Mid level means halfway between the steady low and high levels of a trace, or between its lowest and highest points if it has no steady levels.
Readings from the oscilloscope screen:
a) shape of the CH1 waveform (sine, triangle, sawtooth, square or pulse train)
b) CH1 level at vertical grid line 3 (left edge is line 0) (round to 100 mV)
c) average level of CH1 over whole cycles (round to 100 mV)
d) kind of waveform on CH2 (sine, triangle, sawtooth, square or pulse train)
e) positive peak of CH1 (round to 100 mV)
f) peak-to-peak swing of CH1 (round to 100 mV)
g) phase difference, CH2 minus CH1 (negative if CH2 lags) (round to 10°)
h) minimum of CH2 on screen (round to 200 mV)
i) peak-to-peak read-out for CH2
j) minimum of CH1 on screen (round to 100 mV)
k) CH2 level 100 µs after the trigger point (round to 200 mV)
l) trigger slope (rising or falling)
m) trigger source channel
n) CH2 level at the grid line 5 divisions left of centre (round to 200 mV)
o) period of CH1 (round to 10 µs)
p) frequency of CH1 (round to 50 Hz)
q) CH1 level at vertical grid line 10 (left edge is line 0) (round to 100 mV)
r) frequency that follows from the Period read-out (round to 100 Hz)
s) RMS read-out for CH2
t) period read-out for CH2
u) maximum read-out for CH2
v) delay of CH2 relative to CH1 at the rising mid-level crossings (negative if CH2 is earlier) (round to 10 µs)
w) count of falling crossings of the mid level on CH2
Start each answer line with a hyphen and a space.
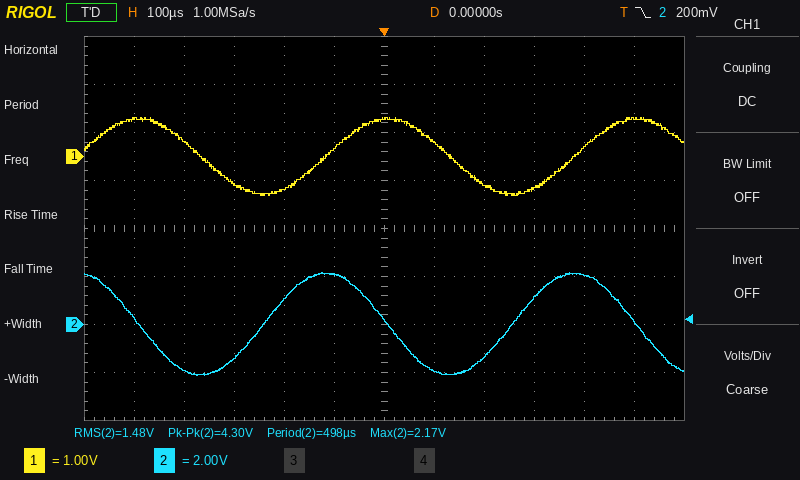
- sine
- -600 mV
- 0.0 V
- sine
- 800 mV
- 1.6 V
- +90°
- -2.2 V
- 4.30 V
- -800 mV
- -2.0 V
- falling
- CH2
- 200 mV
- 500 µs
- 2.00 kHz
- 200 mV
- 2.0 kHz
- 1.48 V
- 498 µs
- 2.17 V
- -120 µs
- 3
